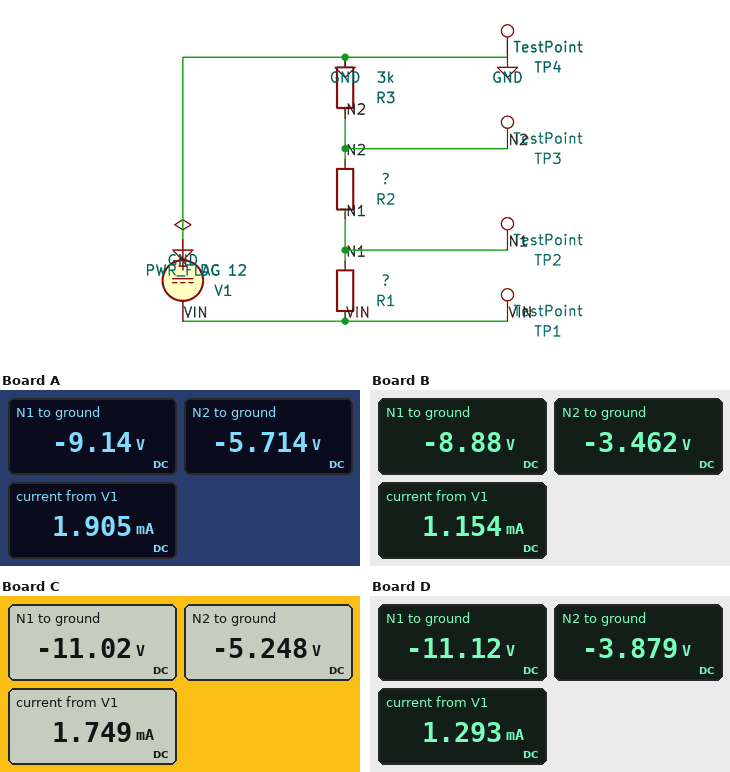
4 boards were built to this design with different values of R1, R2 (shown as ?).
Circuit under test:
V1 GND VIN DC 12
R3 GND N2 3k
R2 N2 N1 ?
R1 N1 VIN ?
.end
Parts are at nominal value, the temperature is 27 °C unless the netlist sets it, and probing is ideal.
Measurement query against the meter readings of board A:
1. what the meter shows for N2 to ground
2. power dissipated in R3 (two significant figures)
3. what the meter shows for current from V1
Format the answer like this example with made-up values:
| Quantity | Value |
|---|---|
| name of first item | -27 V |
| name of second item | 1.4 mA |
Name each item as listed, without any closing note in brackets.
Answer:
| Quantity | Value |
|---|---|
| what the meter shows for N2 to ground | -5.714 V |
| power dissipated in R3 | 11 mW |
| what the meter shows for current from V1 | 1.905 mA |
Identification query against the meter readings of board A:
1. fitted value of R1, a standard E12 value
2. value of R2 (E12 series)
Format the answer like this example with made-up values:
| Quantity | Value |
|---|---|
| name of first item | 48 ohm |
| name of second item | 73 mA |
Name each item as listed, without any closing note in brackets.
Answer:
| Quantity | Value |
|---|---|
| fitted value of R1, a standard E12 value | 1.5 kΩ |
| value of R2 | 1.8 kΩ |
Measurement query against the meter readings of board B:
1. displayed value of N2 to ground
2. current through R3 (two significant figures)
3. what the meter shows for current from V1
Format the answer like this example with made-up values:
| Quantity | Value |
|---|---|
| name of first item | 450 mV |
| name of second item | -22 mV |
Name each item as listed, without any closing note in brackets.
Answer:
| Quantity | Value |
|---|---|
| displayed value of N2 to ground | -3.462 V |
| current through R3 | 1.2 mA |
| what the meter shows for current from V1 | 1.154 mA |
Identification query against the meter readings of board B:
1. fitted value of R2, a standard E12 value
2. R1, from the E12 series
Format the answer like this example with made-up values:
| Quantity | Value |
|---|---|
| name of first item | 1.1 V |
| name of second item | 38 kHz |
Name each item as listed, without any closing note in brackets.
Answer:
| Quantity | Value |
|---|---|
| fitted value of R2, a standard E12 value | 4.7 kΩ |
| R1, from the E12 series | 2.7 kΩ |
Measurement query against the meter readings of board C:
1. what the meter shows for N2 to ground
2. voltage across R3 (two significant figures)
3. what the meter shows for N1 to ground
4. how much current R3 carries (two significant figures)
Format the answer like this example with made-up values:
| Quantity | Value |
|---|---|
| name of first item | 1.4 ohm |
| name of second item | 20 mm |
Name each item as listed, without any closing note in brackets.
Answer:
| Quantity | Value |
|---|---|
| what the meter shows for N2 to ground | -5.248 V |
| voltage across R3 | 5.2 V |
| what the meter shows for N1 to ground | -11.02 V |
| how much current R3 carries | 1.7 mA |
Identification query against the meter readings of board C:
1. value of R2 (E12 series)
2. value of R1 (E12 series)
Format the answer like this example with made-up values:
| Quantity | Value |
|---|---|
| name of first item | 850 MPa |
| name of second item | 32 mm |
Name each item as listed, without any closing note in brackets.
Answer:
| Quantity | Value |
|---|---|
| value of R2 | 3.3 kΩ |
| value of R1 | 560 Ω |
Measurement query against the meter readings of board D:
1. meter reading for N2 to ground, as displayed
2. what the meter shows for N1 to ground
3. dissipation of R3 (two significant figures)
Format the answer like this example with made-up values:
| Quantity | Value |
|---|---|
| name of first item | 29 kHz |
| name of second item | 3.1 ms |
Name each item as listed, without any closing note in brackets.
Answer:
| Quantity | Value |
|---|---|
| meter reading for N2 to ground, as displayed | -3.879 V |
| what the meter shows for N1 to ground | -11.12 V |
| dissipation of R3 | 5.0 mW |
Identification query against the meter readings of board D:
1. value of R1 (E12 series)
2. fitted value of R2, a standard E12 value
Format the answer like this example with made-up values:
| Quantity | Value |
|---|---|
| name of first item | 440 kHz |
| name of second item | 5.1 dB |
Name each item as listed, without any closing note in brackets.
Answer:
| Quantity | Value |
|---|---|
| value of R1 | 680 Ω |
| fitted value of R2, a standard E12 value | 5.6 kΩ |
